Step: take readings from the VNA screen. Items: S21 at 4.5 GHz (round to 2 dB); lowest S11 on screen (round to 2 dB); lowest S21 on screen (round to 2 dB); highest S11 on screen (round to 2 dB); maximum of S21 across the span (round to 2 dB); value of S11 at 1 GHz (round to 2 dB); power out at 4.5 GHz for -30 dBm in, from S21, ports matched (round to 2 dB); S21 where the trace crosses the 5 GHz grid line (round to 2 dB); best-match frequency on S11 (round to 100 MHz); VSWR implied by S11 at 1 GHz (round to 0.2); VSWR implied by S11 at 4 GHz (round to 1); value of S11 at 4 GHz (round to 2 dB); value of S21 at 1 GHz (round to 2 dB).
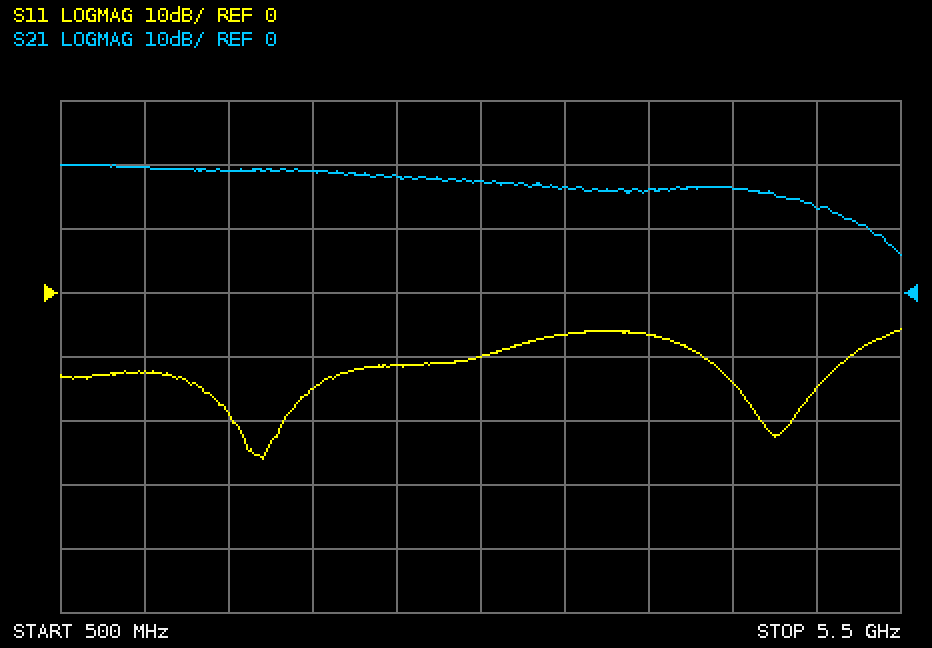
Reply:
16 dB
-26 dB
6 dB
-6 dB
20 dB
-12 dB
-14 dBm
14 dB
1.7 GHz
1.6
3
-6 dB
20 dB
